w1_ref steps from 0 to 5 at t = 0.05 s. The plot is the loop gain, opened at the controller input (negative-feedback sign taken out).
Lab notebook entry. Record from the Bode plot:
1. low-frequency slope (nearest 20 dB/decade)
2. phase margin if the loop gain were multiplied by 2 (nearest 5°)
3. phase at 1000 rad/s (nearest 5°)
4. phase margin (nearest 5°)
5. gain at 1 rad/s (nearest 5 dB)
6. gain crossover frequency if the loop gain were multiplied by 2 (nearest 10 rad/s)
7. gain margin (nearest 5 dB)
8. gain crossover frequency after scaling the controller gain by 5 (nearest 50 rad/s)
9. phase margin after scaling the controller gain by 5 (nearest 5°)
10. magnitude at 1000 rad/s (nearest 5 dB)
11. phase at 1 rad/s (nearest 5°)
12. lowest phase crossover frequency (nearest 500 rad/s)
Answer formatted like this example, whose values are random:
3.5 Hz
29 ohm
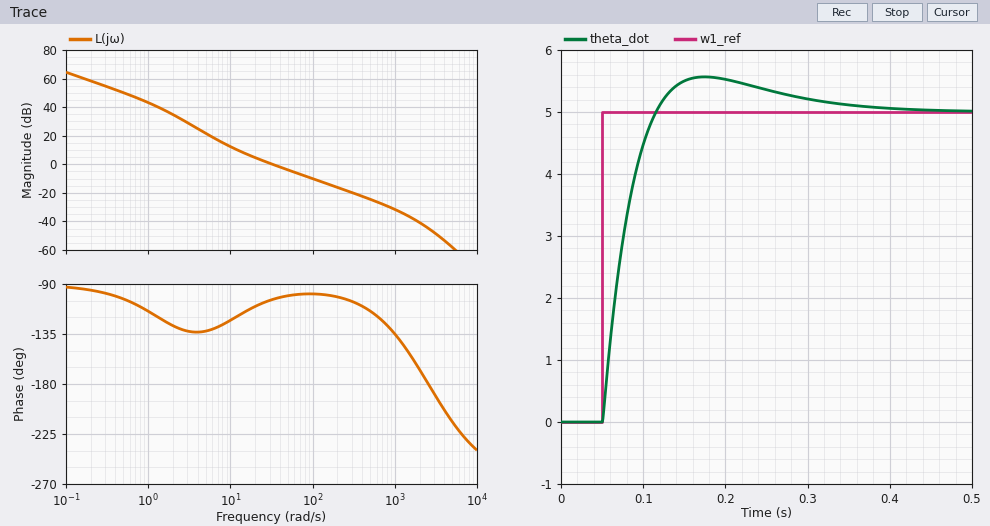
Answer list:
-20 dB/decade
80°
-135°
75°
45 dB
60 rad/s
45 dB
150 rad/s
80°
-30 dB
-115°
2500 rad/s
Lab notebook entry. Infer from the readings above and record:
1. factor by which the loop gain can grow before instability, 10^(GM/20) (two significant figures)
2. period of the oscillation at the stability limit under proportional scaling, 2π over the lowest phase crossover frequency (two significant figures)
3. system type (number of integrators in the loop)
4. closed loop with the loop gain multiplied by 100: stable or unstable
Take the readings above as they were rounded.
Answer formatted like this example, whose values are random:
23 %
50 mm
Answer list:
180
0.0025 s
1
stable
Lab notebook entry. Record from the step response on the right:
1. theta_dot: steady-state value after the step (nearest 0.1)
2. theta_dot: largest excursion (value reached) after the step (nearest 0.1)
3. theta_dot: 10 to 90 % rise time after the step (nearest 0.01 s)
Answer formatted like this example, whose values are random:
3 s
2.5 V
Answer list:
5.0
5.6
0.05 s
